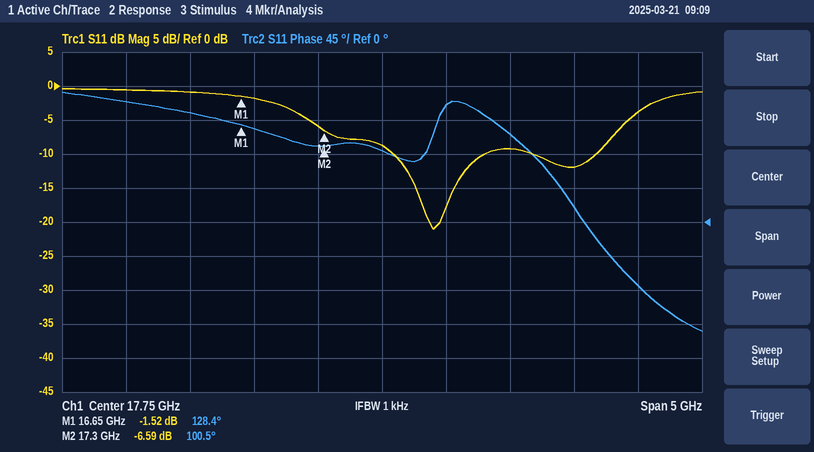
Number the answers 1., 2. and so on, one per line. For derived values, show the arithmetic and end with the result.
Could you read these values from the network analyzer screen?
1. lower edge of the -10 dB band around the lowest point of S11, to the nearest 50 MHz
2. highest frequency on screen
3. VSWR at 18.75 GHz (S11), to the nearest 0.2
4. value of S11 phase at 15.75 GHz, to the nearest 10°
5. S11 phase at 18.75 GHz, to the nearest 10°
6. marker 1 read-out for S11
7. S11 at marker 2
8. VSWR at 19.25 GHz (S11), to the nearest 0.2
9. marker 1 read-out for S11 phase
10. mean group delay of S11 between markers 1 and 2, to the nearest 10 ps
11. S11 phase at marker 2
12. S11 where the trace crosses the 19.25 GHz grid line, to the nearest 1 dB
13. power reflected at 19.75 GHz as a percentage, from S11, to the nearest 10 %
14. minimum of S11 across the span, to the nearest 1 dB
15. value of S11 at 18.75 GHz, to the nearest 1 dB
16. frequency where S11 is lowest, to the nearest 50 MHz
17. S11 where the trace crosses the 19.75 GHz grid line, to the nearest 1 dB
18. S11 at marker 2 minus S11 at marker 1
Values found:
1. 17.85 GHz
2. 20.25 GHz
3. |Γ| = 10^(-9/20) = 0.3548; VSWR = (1 + 0.3548)/(1 − 0.3548) ≈ 2.10, so 2.0 to the nearest 0.2
4. 160°
5. 120°
6. -1.52 dB
7. -6.59 dB
8. |Γ| = 10^(-12/20) = 0.2512; VSWR = (1 + 0.2512)/(1 − 0.2512) ≈ 1.67, so 1.6 to the nearest 0.2
9. 128.4°
10. −(100.5° − (128.4°))/(360° × 650 MHz) ≈ 119 ps, so 120 ps to the nearest 10 ps
11. 100.5°
12. -12 dB
13. 10^(-4/10) ≈ 40 %
14. -21 dB
15. -9 dB
16. 18.15 GHz
17. -4 dB
18. -6.59 − (-1.52) = -5.07 dB
